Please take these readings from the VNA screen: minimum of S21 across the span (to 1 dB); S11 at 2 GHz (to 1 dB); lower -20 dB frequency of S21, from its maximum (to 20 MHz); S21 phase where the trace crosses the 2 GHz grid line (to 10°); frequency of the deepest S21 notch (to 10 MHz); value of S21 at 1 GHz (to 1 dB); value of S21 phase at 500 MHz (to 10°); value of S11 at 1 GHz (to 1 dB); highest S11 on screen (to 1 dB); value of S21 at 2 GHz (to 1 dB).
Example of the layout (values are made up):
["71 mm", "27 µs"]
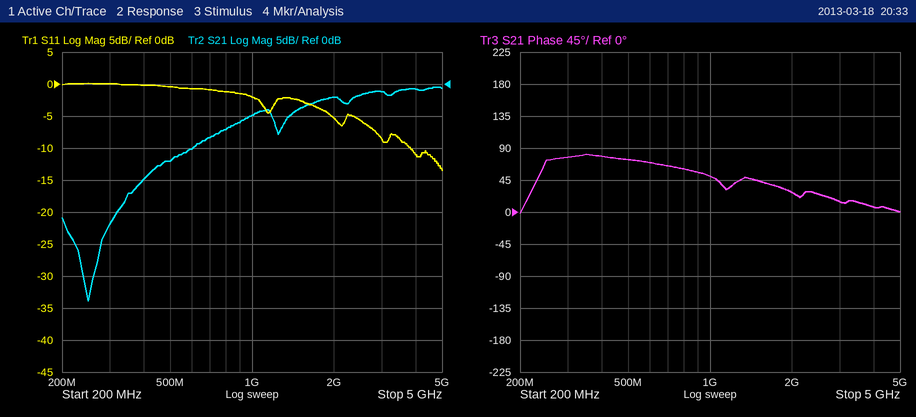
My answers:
["-34 dB", "-5 dB", "320 MHz", "30°", "250 MHz", "-5 dB", "70°", "-2 dB", "0 dB", "-2 dB"]
